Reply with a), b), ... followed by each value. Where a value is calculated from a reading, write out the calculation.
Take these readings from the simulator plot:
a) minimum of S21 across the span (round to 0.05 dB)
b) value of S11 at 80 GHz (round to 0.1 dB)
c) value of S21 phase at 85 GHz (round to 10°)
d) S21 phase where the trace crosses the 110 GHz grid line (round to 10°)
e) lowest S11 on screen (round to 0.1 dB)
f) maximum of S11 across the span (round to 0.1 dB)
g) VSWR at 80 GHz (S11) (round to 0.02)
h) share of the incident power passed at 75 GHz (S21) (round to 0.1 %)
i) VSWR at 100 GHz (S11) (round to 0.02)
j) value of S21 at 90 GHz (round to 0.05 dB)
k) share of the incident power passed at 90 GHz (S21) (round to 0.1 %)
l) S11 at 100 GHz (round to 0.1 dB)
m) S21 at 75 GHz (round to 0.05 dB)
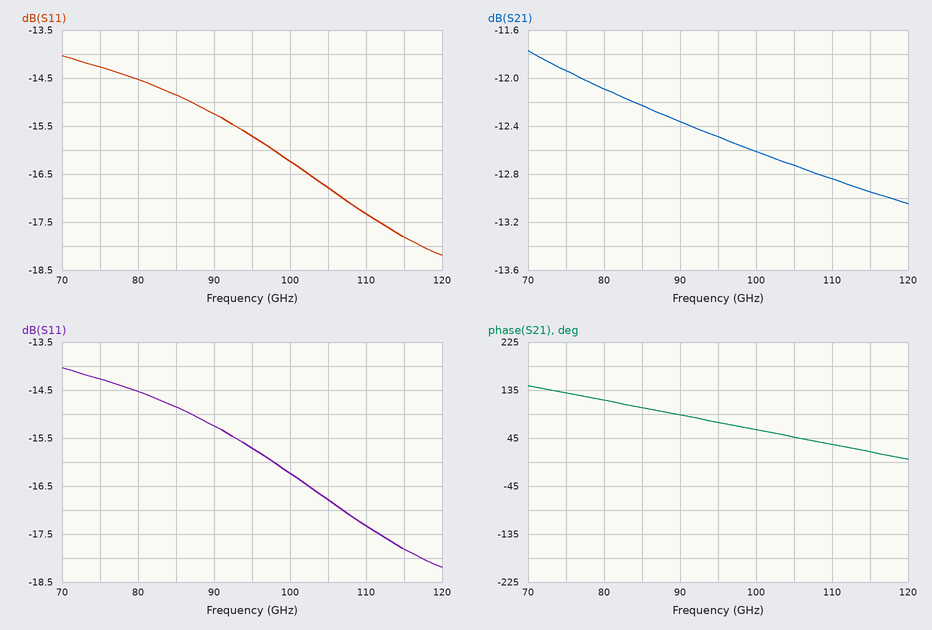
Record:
a) -13.05 dB
b) -14.5 dB
c) 100°
d) 30°
e) -18.2 dB
f) -14.0 dB
g) |Γ| = 10^(-14.5/20) = 0.1884; VSWR = (1 + 0.1884)/(1 − 0.1884) ≈ 1.46
h) 10^(-11.95/10) ≈ 6.4 %
i) |Γ| = 10^(-16.2/20) = 0.1549; VSWR = (1 + 0.1549)/(1 − 0.1549) ≈ 1.37, so 1.36 to the nearest 0.02
j) -12.35 dB
k) 10^(-12.35/10) ≈ 5.8 %
l) -16.2 dB
m) -11.95 dB
